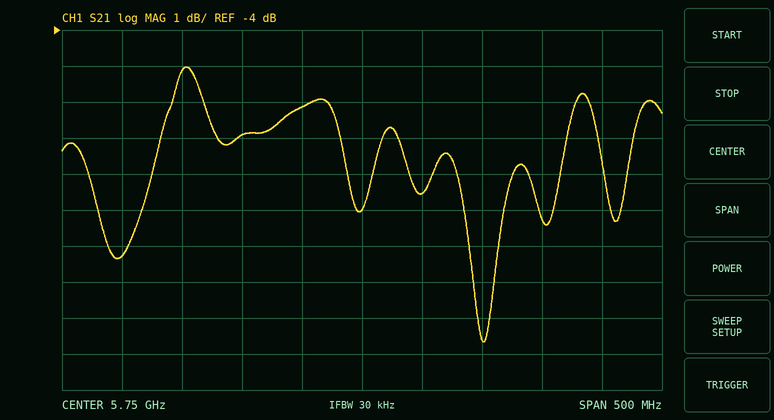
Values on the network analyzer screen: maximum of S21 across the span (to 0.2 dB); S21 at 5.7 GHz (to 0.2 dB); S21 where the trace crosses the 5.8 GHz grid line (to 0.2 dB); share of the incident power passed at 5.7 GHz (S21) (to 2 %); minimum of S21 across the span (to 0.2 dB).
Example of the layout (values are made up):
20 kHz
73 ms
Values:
-5.0 dB
-6.2 dB
-8.6 dB
24 %
-12.6 dB
